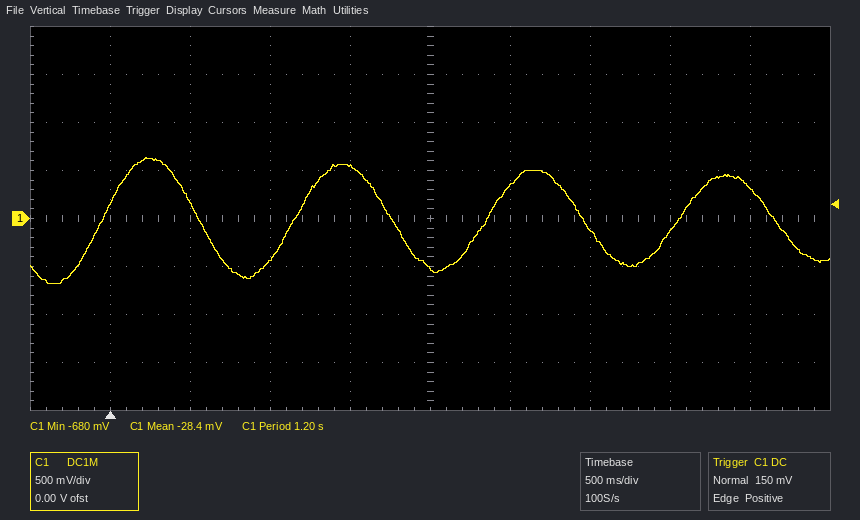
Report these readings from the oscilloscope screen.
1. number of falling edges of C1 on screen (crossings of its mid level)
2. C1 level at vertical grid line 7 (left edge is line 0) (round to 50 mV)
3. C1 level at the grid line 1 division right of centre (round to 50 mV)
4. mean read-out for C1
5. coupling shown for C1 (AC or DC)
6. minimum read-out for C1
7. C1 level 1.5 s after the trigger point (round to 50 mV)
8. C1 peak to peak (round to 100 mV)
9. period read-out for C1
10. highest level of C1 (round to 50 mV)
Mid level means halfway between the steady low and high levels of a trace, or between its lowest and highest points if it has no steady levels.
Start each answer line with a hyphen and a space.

- 4
- -100 mV
- 350 mV
- -28.4 mV
- DC
- -680 mV
- 550 mV
- 1.30 V
- 1.20 s
- 650 mV
